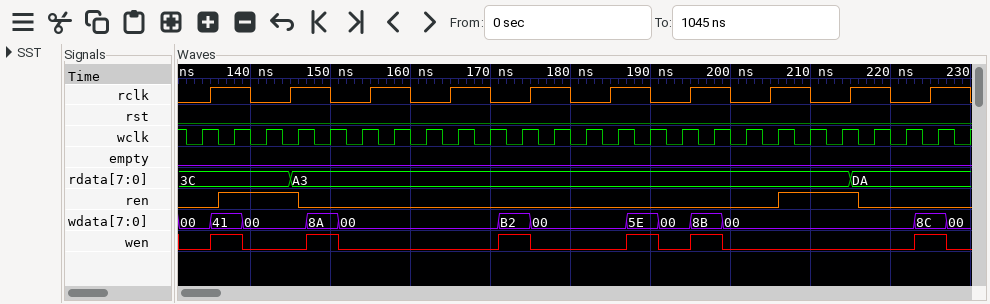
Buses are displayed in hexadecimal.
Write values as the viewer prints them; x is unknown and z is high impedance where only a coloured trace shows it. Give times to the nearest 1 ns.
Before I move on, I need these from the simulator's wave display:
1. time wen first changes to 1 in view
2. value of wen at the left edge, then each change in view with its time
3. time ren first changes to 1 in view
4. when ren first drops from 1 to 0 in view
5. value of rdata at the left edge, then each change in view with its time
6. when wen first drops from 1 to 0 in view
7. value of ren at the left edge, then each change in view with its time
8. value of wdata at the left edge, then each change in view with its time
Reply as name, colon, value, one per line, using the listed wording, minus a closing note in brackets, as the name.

time wen first changes to 1 in view: 135 ns
value of wen at the left edge, then each change in view with its time: 0, 1 at 135 ns, 0 at 139 ns, 1 at 147 ns, 0 at 151 ns, 1 at 171 ns, 0 at 175 ns, 1 at 187 ns, 0 at 191 ns, 1 at 195 ns, 0 at 199 ns, 1 at 223 ns, 0 at 227 ns
time ren first changes to 1 in view: 136 ns
when ren first drops from 1 to 0 in view: 146 ns
value of rdata at the left edge, then each change in view with its time: 3C, A3 at 145 ns, DA at 215 ns
when wen first drops from 1 to 0 in view: 139 ns
value of ren at the left edge, then each change in view with its time: 0, 1 at 136 ns, 0 at 146 ns, 1 at 206 ns, 0 at 216 ns
value of wdata at the left edge, then each change in view with its time: 00, 41 at 135 ns, 00 at 139 ns, 8A at 147 ns, 00 at 151 ns, B2 at 171 ns, 00 at 175 ns, 5E at 187 ns, 00 at 191 ns, 8B at 195 ns, 00 at 199 ns, 8C at 223 ns, 00 at 227 ns
